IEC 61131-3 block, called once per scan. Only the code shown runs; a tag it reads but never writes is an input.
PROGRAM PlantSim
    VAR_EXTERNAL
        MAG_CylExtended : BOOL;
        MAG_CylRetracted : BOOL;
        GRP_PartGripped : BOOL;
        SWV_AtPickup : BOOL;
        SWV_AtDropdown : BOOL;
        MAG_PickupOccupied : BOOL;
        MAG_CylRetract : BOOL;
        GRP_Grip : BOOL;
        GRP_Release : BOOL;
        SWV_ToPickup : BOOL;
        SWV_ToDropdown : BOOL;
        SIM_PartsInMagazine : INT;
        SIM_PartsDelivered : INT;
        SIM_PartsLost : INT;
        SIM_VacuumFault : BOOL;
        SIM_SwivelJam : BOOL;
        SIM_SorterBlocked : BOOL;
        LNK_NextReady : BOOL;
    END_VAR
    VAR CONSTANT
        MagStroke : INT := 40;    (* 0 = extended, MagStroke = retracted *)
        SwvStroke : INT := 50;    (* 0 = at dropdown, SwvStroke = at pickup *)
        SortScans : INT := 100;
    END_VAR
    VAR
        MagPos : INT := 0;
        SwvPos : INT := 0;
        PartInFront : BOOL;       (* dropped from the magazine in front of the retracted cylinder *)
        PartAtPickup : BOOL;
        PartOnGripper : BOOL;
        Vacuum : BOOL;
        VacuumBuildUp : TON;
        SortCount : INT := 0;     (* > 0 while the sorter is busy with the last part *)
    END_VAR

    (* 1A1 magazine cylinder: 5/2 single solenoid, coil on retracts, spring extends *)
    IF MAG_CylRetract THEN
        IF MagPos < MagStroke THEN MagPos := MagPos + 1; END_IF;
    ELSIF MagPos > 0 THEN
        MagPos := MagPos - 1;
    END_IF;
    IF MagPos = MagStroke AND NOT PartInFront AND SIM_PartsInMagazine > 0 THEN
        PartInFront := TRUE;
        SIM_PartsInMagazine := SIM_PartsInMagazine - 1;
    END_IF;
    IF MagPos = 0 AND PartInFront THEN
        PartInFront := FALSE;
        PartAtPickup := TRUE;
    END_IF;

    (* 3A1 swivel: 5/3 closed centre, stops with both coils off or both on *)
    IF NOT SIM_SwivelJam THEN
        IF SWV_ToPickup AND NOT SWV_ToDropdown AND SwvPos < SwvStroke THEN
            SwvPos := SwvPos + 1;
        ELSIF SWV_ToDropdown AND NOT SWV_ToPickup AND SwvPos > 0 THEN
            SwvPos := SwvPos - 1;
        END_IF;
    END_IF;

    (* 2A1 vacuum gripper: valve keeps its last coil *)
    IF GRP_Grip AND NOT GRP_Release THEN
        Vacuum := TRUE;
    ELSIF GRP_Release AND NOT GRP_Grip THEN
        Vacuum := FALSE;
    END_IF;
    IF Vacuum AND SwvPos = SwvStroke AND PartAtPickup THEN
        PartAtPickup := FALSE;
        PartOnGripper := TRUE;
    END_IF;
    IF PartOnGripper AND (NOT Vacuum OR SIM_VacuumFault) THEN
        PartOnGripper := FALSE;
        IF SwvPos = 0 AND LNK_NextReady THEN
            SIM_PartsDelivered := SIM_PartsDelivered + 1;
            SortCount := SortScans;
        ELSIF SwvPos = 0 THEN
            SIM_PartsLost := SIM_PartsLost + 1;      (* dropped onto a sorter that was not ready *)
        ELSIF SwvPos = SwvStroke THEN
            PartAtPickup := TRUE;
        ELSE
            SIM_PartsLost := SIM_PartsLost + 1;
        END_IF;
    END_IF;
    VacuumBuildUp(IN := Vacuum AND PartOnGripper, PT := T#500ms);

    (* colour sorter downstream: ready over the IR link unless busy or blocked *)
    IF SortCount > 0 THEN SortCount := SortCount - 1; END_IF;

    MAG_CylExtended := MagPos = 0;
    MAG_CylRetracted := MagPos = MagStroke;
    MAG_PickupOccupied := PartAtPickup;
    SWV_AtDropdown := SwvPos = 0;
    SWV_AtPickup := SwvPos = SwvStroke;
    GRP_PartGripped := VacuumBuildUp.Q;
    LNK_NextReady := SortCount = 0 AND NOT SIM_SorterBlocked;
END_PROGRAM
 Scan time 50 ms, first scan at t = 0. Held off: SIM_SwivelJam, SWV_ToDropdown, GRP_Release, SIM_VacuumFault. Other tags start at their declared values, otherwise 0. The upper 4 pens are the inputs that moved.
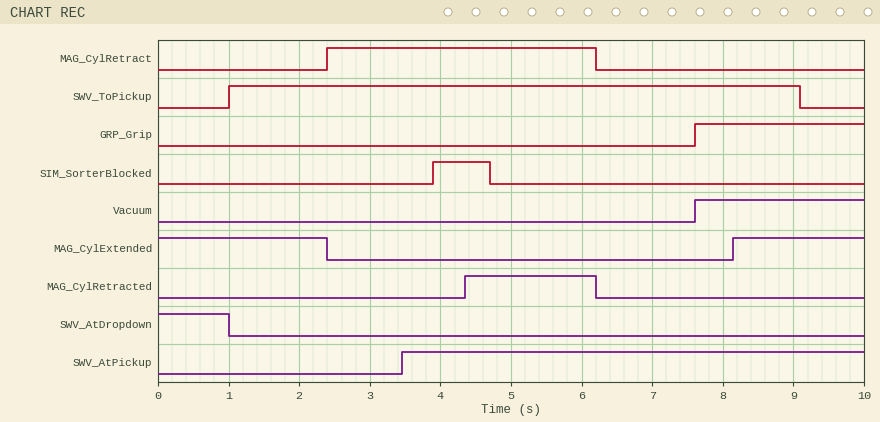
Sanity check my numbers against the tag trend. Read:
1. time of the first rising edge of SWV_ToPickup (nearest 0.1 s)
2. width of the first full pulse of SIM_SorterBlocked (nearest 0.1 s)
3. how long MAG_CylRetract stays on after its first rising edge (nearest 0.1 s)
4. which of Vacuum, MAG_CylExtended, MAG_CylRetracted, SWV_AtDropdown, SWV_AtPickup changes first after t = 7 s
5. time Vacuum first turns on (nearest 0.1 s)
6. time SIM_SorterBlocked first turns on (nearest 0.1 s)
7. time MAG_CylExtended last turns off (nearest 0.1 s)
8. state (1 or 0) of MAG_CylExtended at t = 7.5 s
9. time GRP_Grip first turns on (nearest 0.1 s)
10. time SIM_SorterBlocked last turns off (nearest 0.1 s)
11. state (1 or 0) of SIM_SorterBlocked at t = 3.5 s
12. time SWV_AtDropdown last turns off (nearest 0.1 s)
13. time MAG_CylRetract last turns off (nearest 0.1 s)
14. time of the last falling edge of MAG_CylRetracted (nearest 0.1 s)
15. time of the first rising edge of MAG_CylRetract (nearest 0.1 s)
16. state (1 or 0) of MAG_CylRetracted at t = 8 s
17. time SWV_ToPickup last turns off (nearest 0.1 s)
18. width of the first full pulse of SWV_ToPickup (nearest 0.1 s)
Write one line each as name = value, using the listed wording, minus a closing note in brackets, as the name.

time of the first rising edge of SWV_ToPickup = 1.0 s
width of the first full pulse of SIM_SorterBlocked = 0.8 s
how long MAG_CylRetract stays on after its first rising edge = 3.8 s
which of Vacuum, MAG_CylExtended, MAG_CylRetracted, SWV_AtDropdown, SWV_AtPickup changes first after t = 7 s = Vacuum
time Vacuum first turns on = 7.6 s
time SIM_SorterBlocked first turns on = 3.9 s
time MAG_CylExtended last turns off = 2.4 s
state (1 or 0) of MAG_CylExtended at t = 7.5 s = 0
time GRP_Grip first turns on = 7.6 s
time SIM_SorterBlocked last turns off = 4.7 s
state (1 or 0) of SIM_SorterBlocked at t = 3.5 s = 0
time SWV_AtDropdown last turns off = 1.0 s
time MAG_CylRetract last turns off = 6.2 s
time of the last falling edge of MAG_CylRetracted = 6.2 s
time of the first rising edge of MAG_CylRetract = 2.4 s
state (1 or 0) of MAG_CylRetracted at t = 8 s = 0
time SWV_ToPickup last turns off = 9.1 s
width of the first full pulse of SWV_ToPickup = 8.1 s
